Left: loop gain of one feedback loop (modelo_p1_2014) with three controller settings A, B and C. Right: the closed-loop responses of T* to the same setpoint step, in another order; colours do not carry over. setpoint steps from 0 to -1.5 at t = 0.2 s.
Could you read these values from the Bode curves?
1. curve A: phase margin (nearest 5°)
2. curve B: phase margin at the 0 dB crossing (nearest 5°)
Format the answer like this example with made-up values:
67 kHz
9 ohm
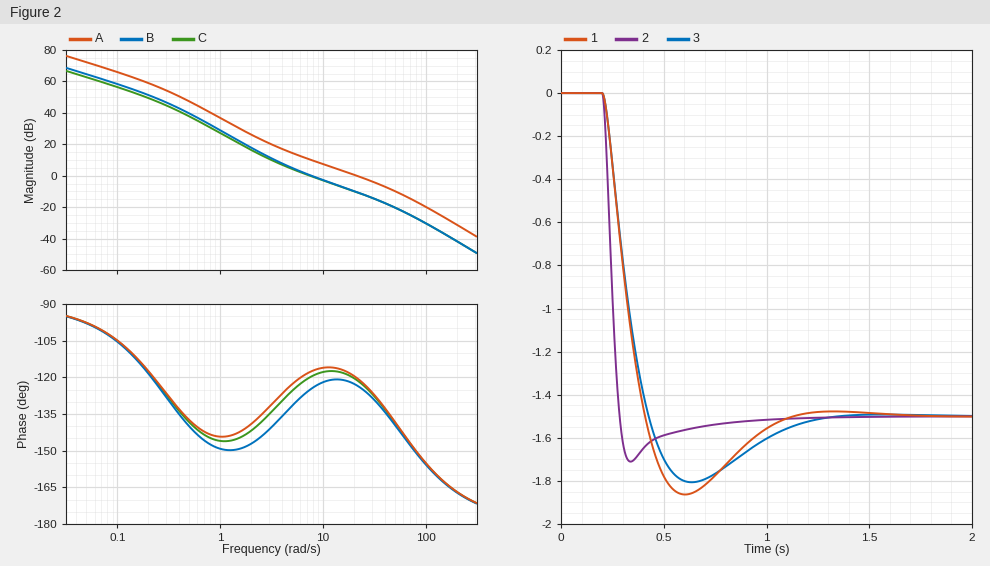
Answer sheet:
60°
55°
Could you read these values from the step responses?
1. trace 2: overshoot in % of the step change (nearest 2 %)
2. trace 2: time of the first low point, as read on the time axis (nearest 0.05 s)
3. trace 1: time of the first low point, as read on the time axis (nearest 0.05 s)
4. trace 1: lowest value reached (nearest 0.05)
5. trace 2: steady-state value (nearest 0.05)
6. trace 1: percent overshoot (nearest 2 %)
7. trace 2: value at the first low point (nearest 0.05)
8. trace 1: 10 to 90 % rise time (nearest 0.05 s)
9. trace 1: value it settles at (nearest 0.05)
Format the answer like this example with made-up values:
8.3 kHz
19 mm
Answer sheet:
14 %
0.35 s
0.60 s
-1.85
-1.50
24 %
-1.70
0.15 s
-1.50
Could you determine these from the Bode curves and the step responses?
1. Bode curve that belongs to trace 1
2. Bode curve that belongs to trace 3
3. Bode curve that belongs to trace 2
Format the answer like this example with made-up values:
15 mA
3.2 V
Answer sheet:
B
C
A
